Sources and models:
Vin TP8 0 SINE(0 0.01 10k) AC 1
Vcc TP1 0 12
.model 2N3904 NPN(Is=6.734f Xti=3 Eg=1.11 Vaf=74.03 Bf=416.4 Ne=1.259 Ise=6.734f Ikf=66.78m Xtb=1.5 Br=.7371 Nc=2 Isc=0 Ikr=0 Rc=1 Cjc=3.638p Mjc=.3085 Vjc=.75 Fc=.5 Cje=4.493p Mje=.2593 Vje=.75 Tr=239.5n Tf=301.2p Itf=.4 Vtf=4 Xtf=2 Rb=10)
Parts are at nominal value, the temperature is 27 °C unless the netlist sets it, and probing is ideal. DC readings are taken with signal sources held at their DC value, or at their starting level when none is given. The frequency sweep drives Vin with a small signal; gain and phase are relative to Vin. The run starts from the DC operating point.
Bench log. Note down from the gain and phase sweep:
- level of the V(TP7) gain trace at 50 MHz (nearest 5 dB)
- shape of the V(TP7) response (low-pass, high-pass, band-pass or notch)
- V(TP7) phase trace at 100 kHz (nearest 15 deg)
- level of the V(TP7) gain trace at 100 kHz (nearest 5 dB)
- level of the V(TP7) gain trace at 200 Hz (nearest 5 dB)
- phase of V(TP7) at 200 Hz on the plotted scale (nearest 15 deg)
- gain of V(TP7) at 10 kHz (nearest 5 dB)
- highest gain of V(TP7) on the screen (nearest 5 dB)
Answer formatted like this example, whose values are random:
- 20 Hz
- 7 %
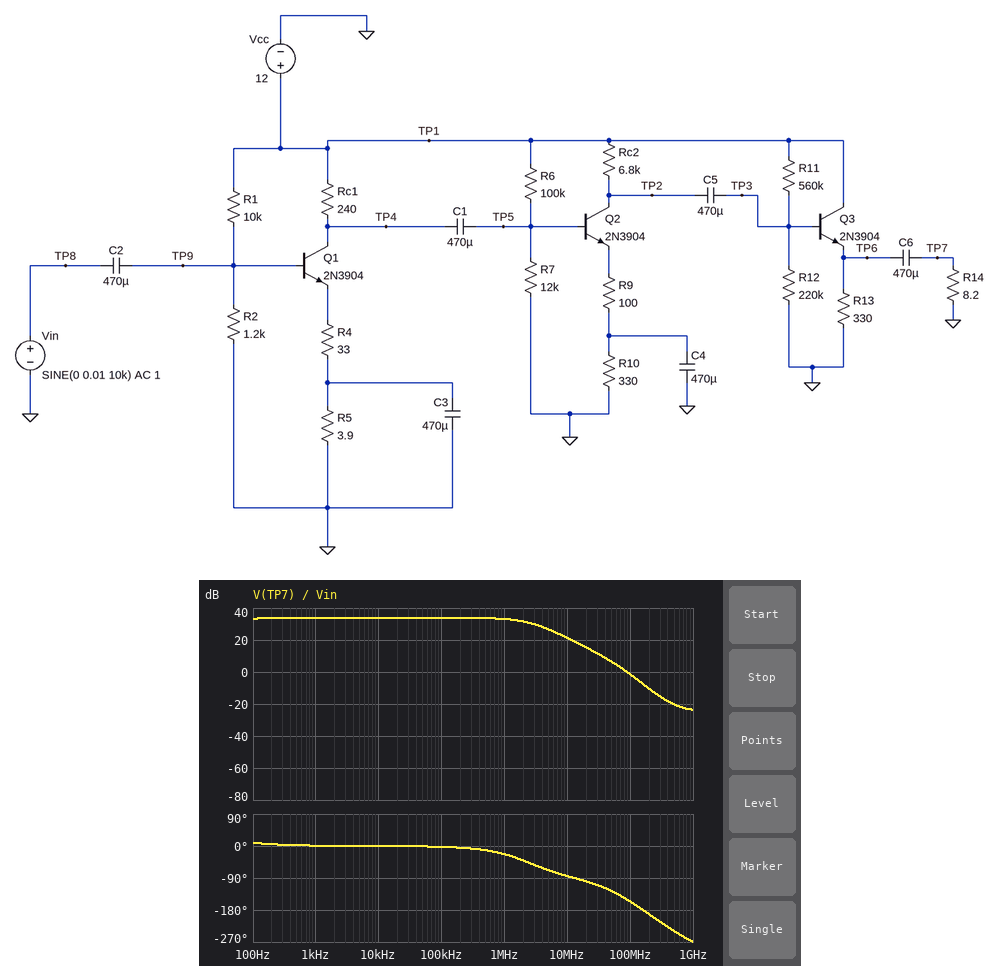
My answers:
- 5 dB
- low-pass
- 0 deg
- 35 dB
- 35 dB
- 0 deg
- 35 dB
- 35 dB
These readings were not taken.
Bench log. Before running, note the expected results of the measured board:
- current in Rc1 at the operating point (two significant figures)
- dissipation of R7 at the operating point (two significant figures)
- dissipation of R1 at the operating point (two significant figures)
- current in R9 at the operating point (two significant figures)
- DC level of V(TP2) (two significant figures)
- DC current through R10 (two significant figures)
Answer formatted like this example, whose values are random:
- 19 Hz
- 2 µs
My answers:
- 13 mA
- 120 µW
- 12 mW
- 1.2 mA
- 3.8 V
- 1.2 mA
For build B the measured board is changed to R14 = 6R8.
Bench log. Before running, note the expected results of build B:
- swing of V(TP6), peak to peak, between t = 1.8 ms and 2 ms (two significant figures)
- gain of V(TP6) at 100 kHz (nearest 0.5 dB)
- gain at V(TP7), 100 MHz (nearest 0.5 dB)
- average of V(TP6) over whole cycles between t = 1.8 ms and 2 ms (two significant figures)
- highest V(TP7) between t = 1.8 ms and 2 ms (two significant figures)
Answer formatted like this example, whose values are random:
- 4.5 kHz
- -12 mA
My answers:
- 410 mV
- 32.5 dB
- -3.0 dB
- 890 mV
- 400 mV
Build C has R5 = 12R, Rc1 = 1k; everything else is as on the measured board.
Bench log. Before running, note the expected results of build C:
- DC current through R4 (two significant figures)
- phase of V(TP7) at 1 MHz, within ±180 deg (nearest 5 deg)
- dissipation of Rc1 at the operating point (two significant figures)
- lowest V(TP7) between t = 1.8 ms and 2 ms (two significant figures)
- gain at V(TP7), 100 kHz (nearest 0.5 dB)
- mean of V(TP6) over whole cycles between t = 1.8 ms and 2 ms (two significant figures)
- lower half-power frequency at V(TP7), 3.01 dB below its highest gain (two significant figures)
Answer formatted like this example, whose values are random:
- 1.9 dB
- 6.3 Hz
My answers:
- 11 mA
- -35 deg
- 110 mW
- -21 mV
- 45.0 dB
- 1.2 V
- 16 Hz
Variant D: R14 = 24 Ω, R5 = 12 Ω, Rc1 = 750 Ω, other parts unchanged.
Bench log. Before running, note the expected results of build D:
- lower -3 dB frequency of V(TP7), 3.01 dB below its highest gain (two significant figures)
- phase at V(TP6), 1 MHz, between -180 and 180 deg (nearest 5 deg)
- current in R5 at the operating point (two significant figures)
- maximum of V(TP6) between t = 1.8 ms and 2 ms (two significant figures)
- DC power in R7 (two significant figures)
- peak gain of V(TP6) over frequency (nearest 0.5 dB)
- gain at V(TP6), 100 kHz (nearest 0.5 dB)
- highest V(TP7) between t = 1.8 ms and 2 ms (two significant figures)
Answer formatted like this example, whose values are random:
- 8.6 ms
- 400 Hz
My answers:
- 14 Hz
- -30 deg
- 11 mA
- 2.9 V
- 120 µW
- 52.0 dB
- 50.0 dB
- 2.1 V
